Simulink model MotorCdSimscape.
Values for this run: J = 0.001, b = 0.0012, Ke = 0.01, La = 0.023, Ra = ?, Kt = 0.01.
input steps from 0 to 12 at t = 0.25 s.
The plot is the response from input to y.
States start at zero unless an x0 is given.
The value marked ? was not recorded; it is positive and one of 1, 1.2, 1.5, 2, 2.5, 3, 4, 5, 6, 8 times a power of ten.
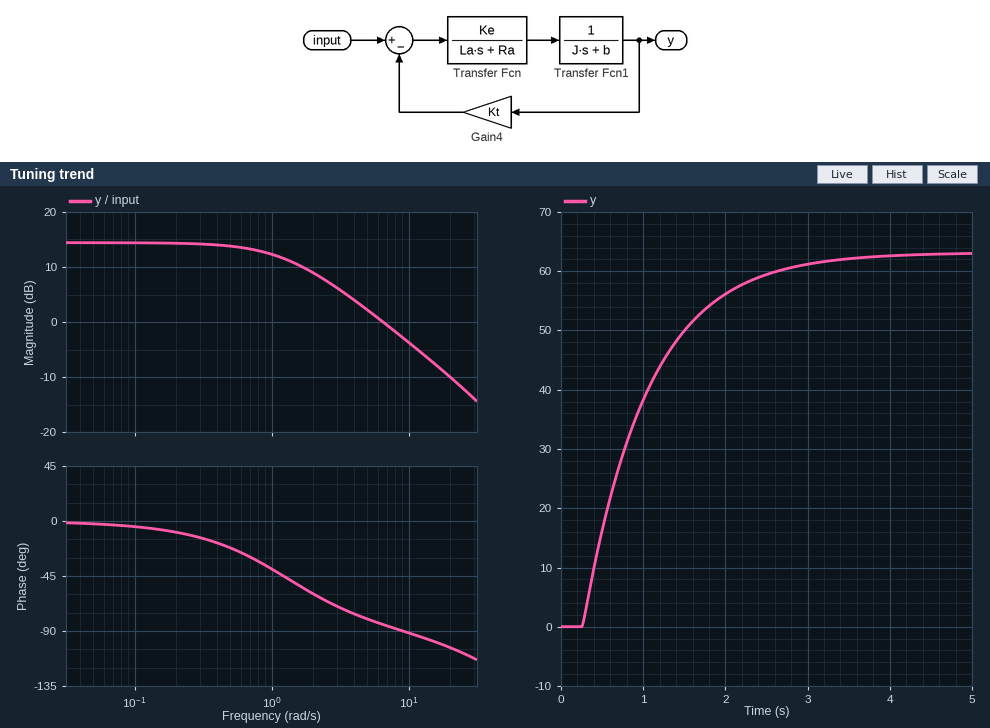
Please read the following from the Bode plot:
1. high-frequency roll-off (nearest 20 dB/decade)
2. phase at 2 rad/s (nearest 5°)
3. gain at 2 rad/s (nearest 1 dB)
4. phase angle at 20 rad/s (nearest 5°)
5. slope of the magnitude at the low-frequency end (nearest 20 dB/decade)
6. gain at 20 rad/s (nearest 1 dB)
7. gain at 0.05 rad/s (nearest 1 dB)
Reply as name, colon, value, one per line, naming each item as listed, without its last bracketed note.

high-frequency roll-off: -20 dB/decade
phase at 2 rad/s: -60°
gain at 2 rad/s: 9 dB
phase angle at 20 rad/s: -105°
slope of the magnitude at the low-frequency end: 0 dB/decade
gain at 20 rad/s: -10 dB
gain at 0.05 rad/s: 14 dB
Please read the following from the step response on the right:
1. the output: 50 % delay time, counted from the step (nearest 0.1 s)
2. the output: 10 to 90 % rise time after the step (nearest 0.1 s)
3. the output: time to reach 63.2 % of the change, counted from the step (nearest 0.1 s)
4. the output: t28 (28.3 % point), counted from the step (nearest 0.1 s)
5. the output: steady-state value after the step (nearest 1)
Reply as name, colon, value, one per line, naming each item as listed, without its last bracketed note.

the output: 50 % delay time, counted from the step: 0.6 s
the output: 10 to 90 % rise time after the step: 1.7 s
the output: time to reach 63.2 % of the change, counted from the step: 0.8 s
the output: t28 (28.3 % point), counted from the step: 0.3 s
the output: steady-state value after the step: 63
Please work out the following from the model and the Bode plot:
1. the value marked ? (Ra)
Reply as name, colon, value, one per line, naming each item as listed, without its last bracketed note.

the value marked ?: 1.5
